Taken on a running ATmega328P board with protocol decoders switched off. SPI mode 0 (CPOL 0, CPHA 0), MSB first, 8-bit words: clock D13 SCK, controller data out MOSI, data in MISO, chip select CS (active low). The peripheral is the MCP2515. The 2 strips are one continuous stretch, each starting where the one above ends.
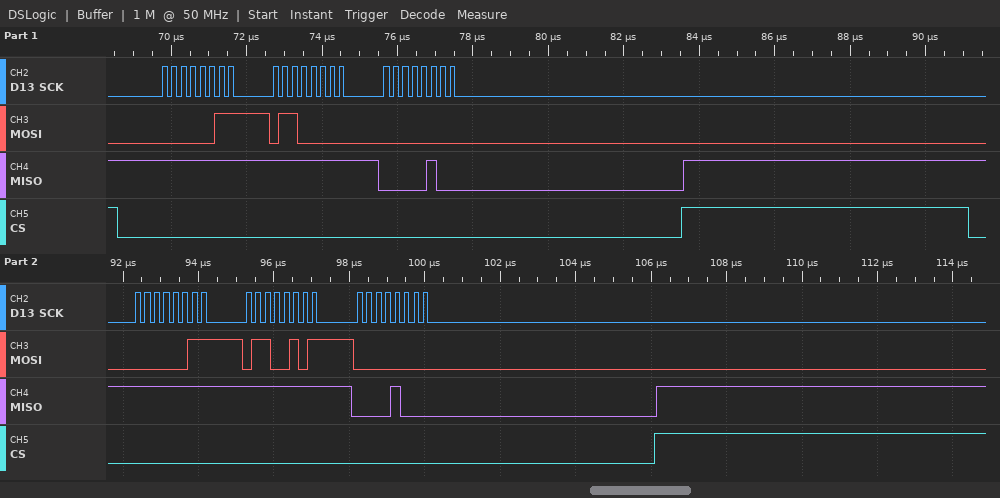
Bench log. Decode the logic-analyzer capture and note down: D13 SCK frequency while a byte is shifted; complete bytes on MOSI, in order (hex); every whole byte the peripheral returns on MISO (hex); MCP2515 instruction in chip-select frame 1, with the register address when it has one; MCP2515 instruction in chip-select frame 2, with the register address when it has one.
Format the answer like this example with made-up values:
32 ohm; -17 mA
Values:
4 MHz; 03 60 00 03 65 00; FF FF 04 FF FF 08; READ 0x60; READ 0x65
